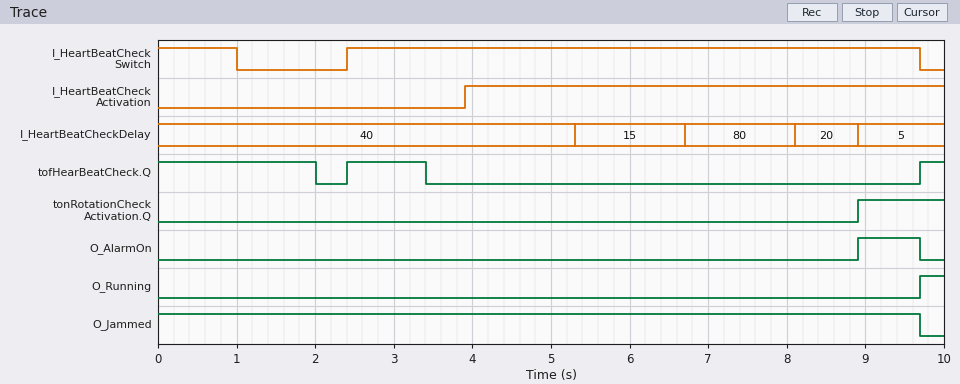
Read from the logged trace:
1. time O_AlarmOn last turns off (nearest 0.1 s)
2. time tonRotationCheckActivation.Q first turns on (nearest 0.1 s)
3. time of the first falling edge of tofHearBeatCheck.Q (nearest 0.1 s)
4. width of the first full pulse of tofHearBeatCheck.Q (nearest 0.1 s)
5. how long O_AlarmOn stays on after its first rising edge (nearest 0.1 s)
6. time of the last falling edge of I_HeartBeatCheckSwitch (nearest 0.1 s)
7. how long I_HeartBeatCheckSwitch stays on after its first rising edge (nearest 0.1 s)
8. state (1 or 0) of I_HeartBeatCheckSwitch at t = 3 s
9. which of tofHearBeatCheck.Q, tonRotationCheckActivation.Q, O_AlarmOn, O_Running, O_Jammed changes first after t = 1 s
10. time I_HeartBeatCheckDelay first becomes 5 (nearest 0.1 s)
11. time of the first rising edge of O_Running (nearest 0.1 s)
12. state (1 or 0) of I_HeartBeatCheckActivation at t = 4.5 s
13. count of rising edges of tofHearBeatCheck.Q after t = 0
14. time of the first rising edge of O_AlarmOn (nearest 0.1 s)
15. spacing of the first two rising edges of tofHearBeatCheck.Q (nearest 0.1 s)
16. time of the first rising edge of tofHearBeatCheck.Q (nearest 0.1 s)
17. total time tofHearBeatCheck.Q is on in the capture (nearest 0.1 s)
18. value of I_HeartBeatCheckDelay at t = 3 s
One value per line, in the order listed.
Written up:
9.7 s
8.9 s
2.0 s
1.0 s
0.8 s
9.7 s
7.3 s
1
tofHearBeatCheck.Q
8.9 s
9.7 s
1
2
8.9 s
7.3 s
2.4 s
3.3 s
40
